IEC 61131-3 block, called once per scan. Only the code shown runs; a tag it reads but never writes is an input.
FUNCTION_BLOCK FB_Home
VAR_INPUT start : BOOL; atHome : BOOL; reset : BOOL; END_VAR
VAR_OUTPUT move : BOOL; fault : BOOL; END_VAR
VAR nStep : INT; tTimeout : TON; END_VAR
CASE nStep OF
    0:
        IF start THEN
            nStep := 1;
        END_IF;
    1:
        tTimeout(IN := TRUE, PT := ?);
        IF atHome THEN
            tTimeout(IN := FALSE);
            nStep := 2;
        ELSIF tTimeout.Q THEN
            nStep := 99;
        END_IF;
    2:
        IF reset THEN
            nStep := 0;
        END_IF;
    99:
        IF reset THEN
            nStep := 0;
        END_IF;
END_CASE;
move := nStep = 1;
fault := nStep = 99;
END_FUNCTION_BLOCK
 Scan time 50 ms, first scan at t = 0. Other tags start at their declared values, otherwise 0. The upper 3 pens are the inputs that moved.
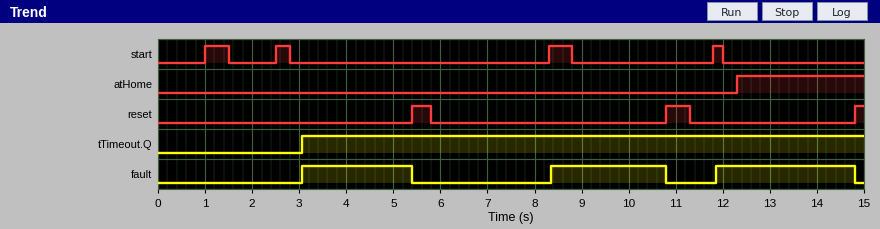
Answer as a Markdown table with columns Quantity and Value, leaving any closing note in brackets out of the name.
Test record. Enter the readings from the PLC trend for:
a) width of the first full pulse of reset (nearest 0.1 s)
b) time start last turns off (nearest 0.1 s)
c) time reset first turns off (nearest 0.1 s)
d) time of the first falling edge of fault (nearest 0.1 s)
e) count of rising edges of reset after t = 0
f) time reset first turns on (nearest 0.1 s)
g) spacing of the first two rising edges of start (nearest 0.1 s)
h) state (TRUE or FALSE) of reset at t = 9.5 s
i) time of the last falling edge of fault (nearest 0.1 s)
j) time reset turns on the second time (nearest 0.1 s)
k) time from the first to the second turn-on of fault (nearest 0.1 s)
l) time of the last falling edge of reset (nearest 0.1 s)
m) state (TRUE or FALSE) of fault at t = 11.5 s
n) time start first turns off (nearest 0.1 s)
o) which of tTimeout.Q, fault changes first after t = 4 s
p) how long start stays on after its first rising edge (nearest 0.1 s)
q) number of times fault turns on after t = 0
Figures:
| Quantity | Value |
|---|---|
| width of the first full pulse of reset | 0.4 s |
| time start last turns off | 12.0 s |
| time reset first turns off | 5.8 s |
| time of the first falling edge of fault | 5.4 s |
| count of rising edges of reset after t = 0 | 3 |
| time reset first turns on | 5.4 s |
| spacing of the first two rising edges of start | 1.5 s |
| state (TRUE or FALSE) of reset at t = 9.5 s | FALSE |
| time of the last falling edge of fault | 14.8 s |
| time reset turns on the second time | 10.8 s |
| time from the first to the second turn-on of fault | 5.3 s |
| time of the last falling edge of reset | 11.3 s |
| state (TRUE or FALSE) of fault at t = 11.5 s | FALSE |
| time start first turns off | 1.5 s |
| which of tTimeout.Q, fault changes first after t = 4 s | fault |
| how long start stays on after its first rising edge | 0.5 s |
| number of times fault turns on after t = 0 | 3 |
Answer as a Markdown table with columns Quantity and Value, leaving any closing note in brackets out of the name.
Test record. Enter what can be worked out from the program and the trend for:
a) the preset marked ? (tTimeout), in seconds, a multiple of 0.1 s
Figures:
| Quantity | Value |
|---|---|
| the preset marked ? (tTimeout), in seconds, a multiple of 0.1 s | 2.0 s |
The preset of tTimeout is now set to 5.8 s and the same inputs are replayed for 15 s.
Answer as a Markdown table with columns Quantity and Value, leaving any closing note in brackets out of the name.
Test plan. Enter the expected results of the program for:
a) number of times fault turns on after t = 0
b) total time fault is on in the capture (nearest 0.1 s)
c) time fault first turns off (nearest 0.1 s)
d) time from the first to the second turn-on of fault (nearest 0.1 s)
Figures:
| Quantity | Value |
|---|---|
| number of times fault turns on after t = 0 | 2 |
| total time fault is on in the capture | 6.9 s |
| time fault first turns off | 10.8 s |
| time from the first to the second turn-on of fault | 5.0 s |
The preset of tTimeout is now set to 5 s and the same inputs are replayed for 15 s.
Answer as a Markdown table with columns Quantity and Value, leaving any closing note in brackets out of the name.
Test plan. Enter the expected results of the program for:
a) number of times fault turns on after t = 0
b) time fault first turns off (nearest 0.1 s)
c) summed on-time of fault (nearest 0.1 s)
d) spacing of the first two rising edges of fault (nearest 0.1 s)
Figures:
| Quantity | Value |
|---|---|
| number of times fault turns on after t = 0 | 2 |
| time fault first turns off | 10.8 s |
| summed on-time of fault | 7.7 s |
| spacing of the first two rising edges of fault | 5.8 s |
